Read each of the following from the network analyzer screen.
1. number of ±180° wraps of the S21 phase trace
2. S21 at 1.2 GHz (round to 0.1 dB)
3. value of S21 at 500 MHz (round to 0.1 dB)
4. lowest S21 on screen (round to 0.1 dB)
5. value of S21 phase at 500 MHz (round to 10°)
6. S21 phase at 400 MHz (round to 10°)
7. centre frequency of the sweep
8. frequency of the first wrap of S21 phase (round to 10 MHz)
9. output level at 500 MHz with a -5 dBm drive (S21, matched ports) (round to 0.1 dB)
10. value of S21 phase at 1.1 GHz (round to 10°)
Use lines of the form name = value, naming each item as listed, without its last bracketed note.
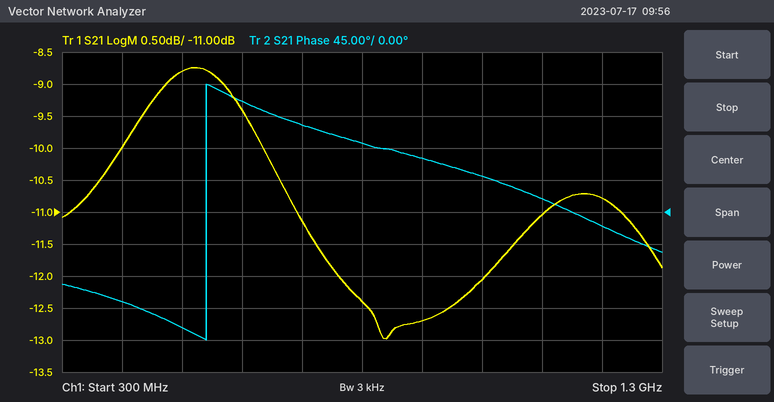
number of ±180° wraps of the S21 phase trace = 1
S21 at 1.2 GHz = -10.8 dB
value of S21 at 500 MHz = -8.8 dB
lowest S21 on screen = -13.0 dB
value of S21 phase at 500 MHz = -160°
S21 phase at 400 MHz = -130°
centre frequency of the sweep = 800 MHz
frequency of the first wrap of S21 phase = 540 MHz
output level at 500 MHz with a -5 dBm drive (S21, matched ports) = -13.8 dBm
value of S21 phase at 1.1 GHz = 20°
